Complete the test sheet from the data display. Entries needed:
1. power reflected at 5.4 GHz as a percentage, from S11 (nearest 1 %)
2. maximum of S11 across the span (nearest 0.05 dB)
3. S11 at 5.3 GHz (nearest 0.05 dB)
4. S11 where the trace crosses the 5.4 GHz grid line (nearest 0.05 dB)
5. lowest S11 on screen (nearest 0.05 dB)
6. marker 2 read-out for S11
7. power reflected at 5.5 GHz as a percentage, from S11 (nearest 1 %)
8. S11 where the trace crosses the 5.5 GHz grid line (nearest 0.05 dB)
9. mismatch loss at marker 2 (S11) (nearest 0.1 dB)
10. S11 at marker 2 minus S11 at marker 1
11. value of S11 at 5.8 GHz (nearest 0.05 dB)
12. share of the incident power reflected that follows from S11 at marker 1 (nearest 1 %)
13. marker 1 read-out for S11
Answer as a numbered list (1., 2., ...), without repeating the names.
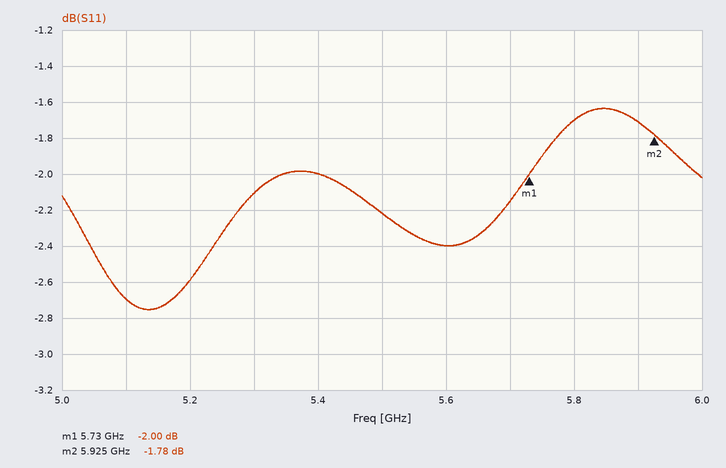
1. 63 %
2. -1.65 dB
3. -2.10 dB
4. -2.00 dB
5. -2.75 dB
6. -1.78 dB
7. 60 %
8. -2.20 dB
9. 4.7 dB
10. 0.22 dB
11. -1.70 dB
12. 63 %
13. -2.00 dB
